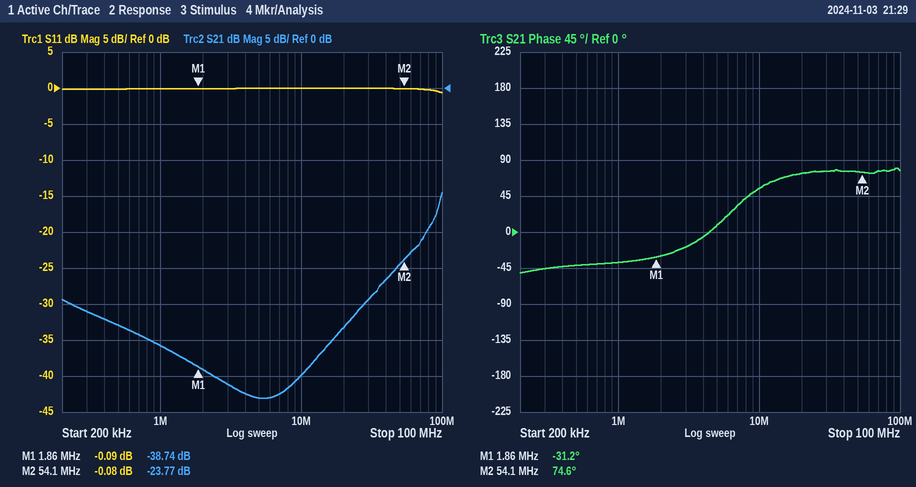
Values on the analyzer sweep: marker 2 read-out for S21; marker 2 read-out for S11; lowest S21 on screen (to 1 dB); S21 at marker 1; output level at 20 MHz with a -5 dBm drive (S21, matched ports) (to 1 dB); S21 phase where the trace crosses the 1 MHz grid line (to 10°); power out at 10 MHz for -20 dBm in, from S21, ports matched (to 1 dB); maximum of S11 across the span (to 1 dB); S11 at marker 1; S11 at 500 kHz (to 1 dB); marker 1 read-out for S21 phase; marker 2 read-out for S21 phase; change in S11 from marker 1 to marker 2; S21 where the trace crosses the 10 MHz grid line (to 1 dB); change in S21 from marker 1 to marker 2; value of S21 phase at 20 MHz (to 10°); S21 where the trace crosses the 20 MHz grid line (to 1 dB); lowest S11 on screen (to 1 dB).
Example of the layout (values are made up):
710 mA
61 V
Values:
-23.77 dB
-0.08 dB
-43 dB
-38.74 dB
-38 dBm
-40°
-60 dBm
0 dB
-0.09 dB
0 dB
-31.2°
74.6°
0.01 dB
-40 dB
14.97 dB
70°
-33 dB
-1 dB
